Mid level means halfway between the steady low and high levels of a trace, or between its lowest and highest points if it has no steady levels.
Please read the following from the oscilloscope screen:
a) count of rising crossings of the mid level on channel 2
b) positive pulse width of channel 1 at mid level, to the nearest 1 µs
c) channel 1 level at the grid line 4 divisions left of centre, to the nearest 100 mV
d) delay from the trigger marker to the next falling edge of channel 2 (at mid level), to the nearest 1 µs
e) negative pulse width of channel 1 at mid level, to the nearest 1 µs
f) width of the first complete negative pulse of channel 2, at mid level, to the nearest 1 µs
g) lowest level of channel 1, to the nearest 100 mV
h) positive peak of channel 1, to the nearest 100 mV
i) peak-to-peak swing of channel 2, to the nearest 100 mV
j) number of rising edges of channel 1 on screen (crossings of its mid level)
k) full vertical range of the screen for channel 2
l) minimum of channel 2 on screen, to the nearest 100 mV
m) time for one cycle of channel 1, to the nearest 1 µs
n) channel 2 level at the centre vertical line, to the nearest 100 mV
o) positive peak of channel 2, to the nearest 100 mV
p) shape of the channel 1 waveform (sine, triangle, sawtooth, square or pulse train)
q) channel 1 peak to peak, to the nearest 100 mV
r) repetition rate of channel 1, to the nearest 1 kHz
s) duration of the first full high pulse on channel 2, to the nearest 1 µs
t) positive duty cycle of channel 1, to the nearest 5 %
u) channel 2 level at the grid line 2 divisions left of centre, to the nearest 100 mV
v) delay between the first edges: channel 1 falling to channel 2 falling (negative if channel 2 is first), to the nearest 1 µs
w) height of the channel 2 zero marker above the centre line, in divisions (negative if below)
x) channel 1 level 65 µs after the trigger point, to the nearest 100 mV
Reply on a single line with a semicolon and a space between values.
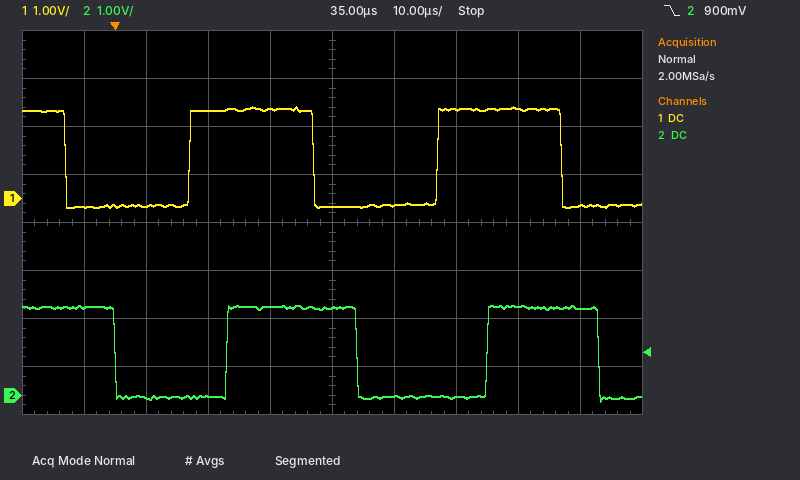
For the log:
2; 20 µs; -200 mV; 39 µs; 20 µs; 18 µs; -200 mV; 1.9 V; 2.0 V; 2; 8 V; -100 mV; 40 µs; 1.8 V; 1.9 V; square; 2.1 V; 25 kHz; 21 µs; 50 %; 0.0 V; +8 µs; -3.6 div; 1.9 V
